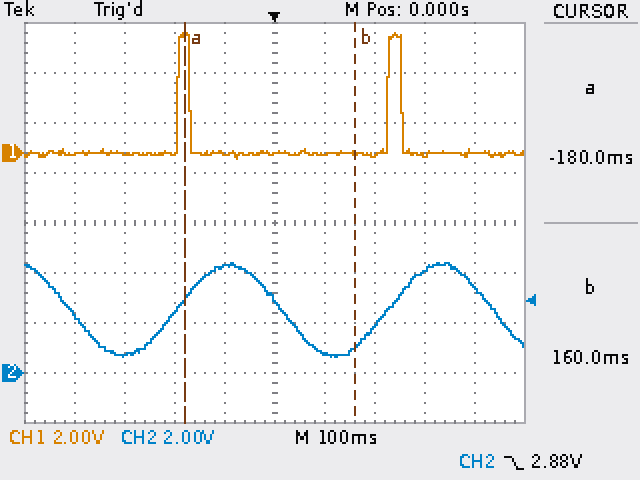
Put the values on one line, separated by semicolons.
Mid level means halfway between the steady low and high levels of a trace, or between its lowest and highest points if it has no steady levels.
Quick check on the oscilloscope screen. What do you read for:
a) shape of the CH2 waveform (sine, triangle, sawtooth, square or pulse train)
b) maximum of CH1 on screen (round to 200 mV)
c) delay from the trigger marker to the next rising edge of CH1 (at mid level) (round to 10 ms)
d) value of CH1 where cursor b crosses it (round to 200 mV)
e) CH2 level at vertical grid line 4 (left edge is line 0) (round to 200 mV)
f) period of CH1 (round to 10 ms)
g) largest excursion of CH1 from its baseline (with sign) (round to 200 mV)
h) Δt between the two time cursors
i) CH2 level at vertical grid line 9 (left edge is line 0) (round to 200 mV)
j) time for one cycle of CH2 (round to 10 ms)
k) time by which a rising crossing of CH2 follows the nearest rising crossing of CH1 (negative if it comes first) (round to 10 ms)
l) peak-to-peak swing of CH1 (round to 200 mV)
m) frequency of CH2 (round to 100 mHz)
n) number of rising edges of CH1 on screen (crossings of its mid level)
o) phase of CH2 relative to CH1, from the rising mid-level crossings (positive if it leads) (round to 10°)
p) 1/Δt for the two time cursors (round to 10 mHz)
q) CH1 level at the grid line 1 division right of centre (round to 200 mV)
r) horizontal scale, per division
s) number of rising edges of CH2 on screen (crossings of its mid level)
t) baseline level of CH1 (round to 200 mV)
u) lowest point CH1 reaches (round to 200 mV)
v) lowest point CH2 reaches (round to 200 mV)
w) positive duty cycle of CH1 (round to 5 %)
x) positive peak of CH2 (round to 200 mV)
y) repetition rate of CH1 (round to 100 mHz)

sine; 4.8 V; 230 ms; 0.0 V; 4.2 V; 420 ms; +4.8 V; 340 ms; 3.4 V; 420 ms; 0 ms; 5.0 V; 2.4 Hz; 2; 0°; 2.94 Hz; 0.0 V; 100 ms; 2; 0.0 V; -200 mV; 600 mV; 5 %; 4.4 V; 2.4 Hz
